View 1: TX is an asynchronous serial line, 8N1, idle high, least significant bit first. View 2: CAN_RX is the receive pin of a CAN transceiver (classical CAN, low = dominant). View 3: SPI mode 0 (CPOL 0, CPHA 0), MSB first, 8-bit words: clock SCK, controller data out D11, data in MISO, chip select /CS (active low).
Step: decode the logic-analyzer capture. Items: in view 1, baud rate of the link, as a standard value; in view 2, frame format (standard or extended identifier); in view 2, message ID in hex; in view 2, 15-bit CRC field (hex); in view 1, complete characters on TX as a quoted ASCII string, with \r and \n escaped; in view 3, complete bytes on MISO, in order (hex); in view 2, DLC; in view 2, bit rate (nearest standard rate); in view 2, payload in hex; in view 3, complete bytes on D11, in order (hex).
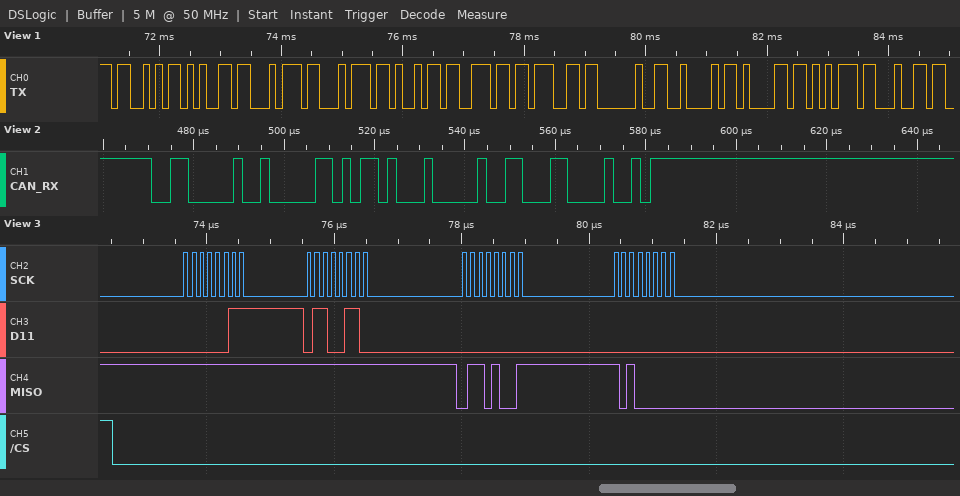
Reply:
9600 baud
standard
0x301
0x3184
"Setting Baud"
0xFF 0xFF 0x69 0xA0
2
500 kbit/s
B4 40
0x03 0x66 0x00 0x00
